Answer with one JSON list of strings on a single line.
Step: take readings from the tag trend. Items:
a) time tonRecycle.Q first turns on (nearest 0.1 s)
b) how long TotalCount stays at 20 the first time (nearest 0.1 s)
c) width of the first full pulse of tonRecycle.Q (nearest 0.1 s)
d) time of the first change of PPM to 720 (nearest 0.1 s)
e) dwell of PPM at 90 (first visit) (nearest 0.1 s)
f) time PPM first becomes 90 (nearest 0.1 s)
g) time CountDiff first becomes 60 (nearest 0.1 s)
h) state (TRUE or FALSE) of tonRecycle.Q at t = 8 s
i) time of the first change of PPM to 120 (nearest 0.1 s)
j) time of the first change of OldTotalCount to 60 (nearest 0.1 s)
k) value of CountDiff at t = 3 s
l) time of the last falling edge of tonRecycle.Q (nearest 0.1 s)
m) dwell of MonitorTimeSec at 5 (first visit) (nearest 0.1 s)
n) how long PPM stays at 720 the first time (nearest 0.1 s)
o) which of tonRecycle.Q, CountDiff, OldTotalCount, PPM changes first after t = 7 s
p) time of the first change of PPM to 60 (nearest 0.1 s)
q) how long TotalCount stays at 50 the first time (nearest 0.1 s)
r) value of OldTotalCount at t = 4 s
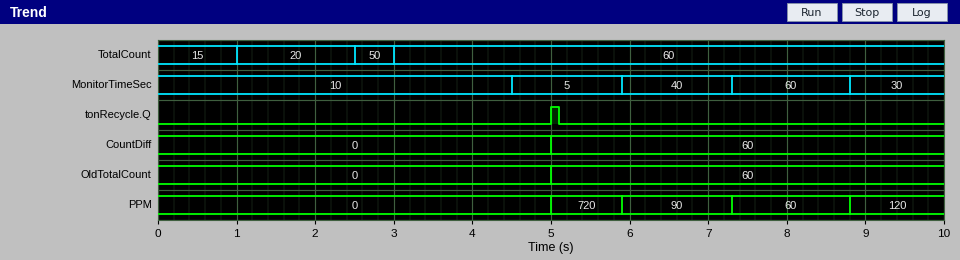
["5.0 s", "1.5 s", "0.1 s", "5.0 s", "1.4 s", "5.9 s", "5.0 s", "FALSE", "8.8 s", "5.0 s", "0", "5.1 s", "1.4 s", "0.9 s", "PPM", "7.3 s", "0.5 s", "0"]
